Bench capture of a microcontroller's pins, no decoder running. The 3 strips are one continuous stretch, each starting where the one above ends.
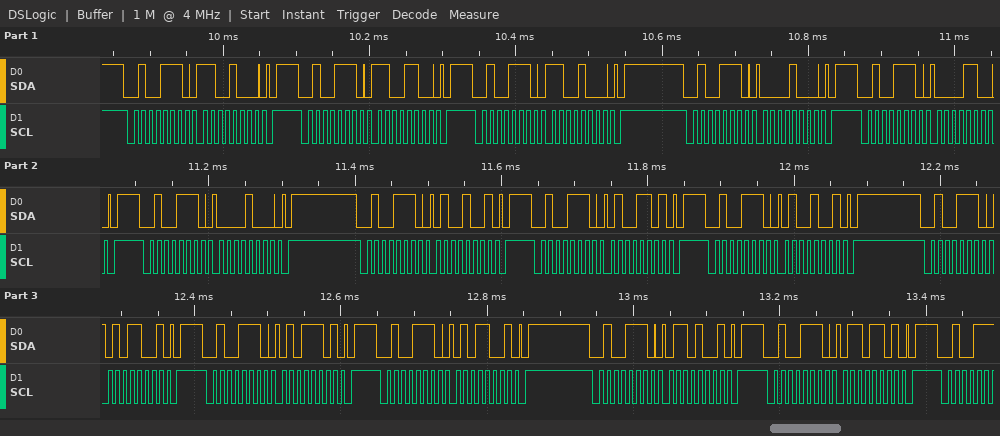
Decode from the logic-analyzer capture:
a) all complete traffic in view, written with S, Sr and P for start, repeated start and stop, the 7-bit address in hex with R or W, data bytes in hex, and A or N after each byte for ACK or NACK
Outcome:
S 27W A C8 A P S 27W A CC A P S 27W A C8 A P S 27W A 08 A P S 27W A 0C A P S 27W A 08 A P S 27W A 49 A P S 27W A 4D A P S 27W A 49 A P S 27W A 59 A P S 27W A 5D A P S 27W A 59 A P S 27W A 69 A P S 27W A 6D A P
